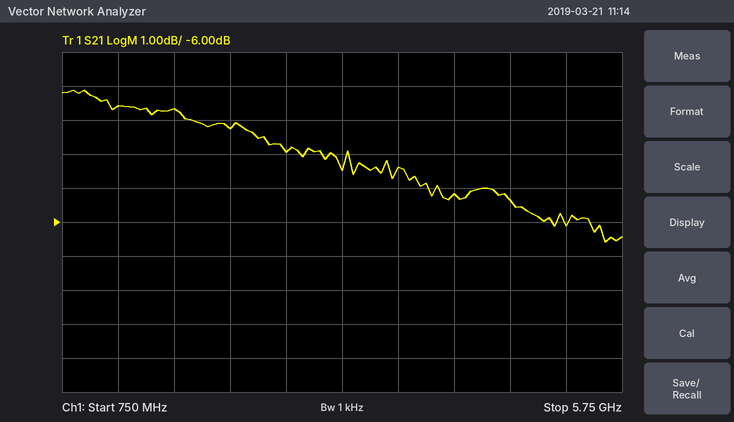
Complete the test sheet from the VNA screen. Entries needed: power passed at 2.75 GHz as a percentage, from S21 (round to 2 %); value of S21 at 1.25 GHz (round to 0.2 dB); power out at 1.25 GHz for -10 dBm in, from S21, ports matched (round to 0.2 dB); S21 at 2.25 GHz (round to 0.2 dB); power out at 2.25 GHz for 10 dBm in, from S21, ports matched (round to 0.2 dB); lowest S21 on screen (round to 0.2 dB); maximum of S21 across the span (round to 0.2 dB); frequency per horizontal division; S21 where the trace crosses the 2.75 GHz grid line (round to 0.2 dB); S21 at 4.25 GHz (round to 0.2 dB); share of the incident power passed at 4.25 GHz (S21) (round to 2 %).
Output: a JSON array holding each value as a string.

["40 %", "-2.6 dB", "-12.6 dBm", "-3.2 dB", "6.8 dBm", "-6.6 dB", "-2.2 dB", "500 MHz", "-4.0 dB", "-5.2 dB", "30 %"]
